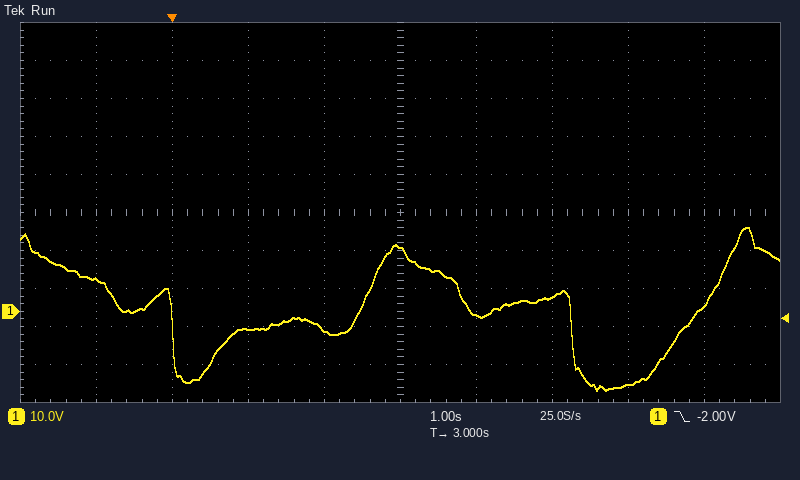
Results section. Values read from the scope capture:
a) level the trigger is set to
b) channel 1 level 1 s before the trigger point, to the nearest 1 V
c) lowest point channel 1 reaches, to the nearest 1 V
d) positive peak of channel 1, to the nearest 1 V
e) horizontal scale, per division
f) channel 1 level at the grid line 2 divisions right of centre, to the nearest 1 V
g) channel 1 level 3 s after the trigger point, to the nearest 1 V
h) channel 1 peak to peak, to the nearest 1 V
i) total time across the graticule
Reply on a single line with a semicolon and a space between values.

-2.00 V; 8 V; -21 V; 22 V; 1 s; 4 V; 17 V; 43 V; 10 s
